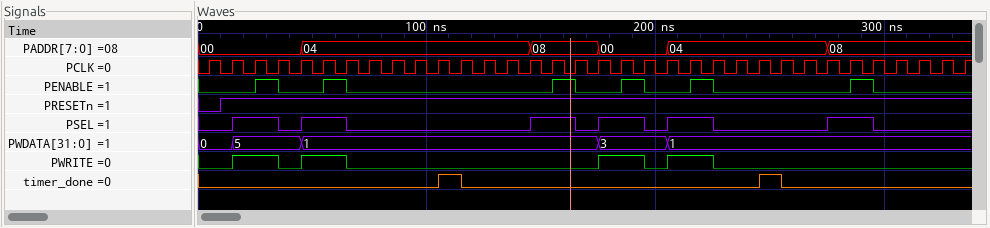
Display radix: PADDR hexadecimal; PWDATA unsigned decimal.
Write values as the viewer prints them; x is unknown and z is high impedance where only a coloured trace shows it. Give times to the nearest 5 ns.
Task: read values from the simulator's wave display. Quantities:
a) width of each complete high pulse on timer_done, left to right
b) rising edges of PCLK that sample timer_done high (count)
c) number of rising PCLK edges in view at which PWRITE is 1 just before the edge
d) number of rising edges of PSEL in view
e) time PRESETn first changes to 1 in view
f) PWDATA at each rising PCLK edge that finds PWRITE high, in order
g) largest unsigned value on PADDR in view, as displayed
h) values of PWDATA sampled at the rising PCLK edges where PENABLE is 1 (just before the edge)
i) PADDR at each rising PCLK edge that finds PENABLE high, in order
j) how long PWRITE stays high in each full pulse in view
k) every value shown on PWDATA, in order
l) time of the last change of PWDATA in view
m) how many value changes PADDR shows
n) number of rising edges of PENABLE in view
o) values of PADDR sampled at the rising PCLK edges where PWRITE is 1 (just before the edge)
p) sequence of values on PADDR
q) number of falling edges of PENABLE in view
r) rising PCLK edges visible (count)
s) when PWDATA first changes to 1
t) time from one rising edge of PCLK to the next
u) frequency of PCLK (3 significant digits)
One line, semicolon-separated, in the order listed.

10 ns, 10 ns; 2; 8; 6; 10 ns; 5, 5, 1, 1, 3, 3, 1, 1; 08; 5, 1, 1, 3, 1, 1; 00, 04, 08, 00, 04, 08; 20 ns, 20 ns, 20 ns, 20 ns; 0, 5, 1, 3, 1; 205 ns; 5; 6; 00, 00, 04, 04, 00, 00, 04, 04; 00, 04, 08, 00, 04, 08; 6; 34; 45 ns; 10 ns; 100 MHz
